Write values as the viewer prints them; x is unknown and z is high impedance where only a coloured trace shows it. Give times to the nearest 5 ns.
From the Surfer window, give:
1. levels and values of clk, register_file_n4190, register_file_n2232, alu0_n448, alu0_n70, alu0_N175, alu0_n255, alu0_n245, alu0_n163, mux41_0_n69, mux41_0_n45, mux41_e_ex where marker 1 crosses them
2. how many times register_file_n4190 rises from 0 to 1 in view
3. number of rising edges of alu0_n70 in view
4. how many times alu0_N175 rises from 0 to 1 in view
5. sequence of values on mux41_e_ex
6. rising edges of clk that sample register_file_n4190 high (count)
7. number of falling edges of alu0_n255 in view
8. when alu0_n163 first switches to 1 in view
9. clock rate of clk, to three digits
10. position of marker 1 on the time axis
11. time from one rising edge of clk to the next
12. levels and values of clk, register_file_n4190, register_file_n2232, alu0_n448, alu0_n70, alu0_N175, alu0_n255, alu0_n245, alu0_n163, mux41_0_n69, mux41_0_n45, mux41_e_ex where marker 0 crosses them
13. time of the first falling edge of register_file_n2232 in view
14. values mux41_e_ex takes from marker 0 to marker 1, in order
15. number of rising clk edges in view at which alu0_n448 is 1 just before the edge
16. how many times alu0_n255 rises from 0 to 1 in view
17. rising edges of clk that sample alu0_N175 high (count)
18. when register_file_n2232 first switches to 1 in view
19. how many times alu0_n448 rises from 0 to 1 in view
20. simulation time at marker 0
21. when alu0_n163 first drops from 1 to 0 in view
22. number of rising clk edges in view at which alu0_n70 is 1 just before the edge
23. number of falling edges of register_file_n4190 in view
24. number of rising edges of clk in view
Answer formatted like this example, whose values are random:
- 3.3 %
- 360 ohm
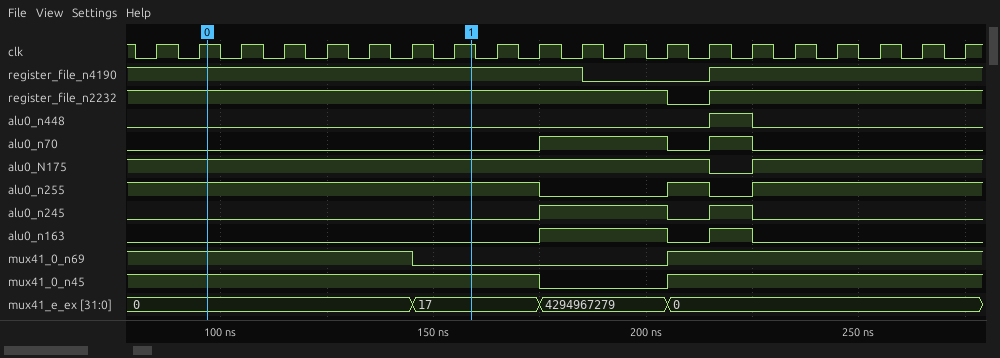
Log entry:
- clk=1, register_file_n4190=1, register_file_n2232=1, alu0_n448=0, alu0_n70=0, alu0_N175=1, alu0_n255=1, alu0_n245=0, alu0_n163=0, mux41_0_n69=0, mux41_0_n45=1, mux41_e_ex=17
- 1
- 2
- 1
- 0, 17, 4294967279, 0
- 17
- 2
- 175 ns
- 100 MHz
- 160 ns
- 10 ns
- clk=1, register_file_n4190=1, register_file_n2232=1, alu0_n448=0, alu0_n70=0, alu0_N175=1, alu0_n255=1, alu0_n245=0, alu0_n163=0, mux41_0_n69=1, mux41_0_n45=1, mux41_e_ex=0
- 205 ns
- 0, 17
- 1
- 2
- 19
- 215 ns
- 1
- 95 ns
- 205 ns
- 4
- 1
- 20
